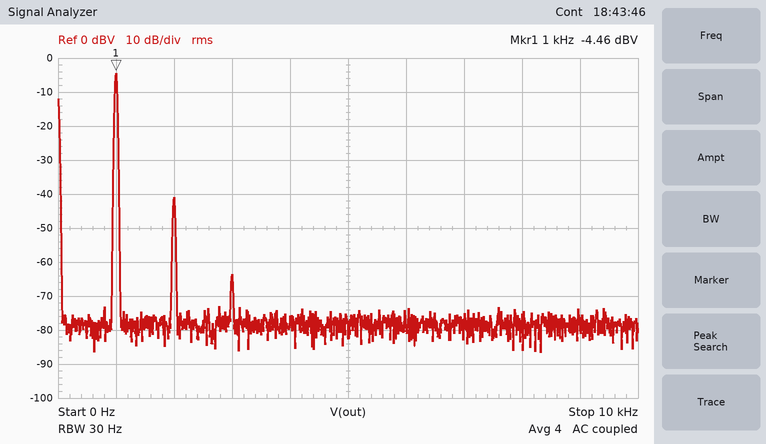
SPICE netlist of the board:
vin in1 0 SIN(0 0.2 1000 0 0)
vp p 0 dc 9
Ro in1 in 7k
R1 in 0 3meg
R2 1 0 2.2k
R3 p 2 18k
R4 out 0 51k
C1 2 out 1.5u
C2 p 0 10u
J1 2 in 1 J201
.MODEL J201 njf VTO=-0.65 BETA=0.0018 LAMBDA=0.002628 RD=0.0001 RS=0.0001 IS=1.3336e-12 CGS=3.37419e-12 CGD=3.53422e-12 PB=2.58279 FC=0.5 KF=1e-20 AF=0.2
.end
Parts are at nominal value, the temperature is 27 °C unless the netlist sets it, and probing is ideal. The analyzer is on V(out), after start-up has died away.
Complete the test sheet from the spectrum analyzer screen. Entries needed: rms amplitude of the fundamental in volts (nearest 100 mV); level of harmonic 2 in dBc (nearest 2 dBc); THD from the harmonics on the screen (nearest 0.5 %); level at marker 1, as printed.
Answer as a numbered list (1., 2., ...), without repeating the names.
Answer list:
1. 600 mV
2. -36 dBc
3. 1.5 %
4. -4.46 dBV
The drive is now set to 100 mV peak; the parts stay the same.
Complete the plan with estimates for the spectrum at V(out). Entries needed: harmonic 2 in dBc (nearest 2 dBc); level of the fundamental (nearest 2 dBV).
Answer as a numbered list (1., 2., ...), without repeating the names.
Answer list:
1. -42 dBc
2. -10 dBV
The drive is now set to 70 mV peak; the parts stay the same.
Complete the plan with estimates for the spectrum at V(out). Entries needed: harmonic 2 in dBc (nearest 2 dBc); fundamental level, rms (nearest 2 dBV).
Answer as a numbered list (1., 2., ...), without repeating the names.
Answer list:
1. -46 dBc
2. -14 dBV
